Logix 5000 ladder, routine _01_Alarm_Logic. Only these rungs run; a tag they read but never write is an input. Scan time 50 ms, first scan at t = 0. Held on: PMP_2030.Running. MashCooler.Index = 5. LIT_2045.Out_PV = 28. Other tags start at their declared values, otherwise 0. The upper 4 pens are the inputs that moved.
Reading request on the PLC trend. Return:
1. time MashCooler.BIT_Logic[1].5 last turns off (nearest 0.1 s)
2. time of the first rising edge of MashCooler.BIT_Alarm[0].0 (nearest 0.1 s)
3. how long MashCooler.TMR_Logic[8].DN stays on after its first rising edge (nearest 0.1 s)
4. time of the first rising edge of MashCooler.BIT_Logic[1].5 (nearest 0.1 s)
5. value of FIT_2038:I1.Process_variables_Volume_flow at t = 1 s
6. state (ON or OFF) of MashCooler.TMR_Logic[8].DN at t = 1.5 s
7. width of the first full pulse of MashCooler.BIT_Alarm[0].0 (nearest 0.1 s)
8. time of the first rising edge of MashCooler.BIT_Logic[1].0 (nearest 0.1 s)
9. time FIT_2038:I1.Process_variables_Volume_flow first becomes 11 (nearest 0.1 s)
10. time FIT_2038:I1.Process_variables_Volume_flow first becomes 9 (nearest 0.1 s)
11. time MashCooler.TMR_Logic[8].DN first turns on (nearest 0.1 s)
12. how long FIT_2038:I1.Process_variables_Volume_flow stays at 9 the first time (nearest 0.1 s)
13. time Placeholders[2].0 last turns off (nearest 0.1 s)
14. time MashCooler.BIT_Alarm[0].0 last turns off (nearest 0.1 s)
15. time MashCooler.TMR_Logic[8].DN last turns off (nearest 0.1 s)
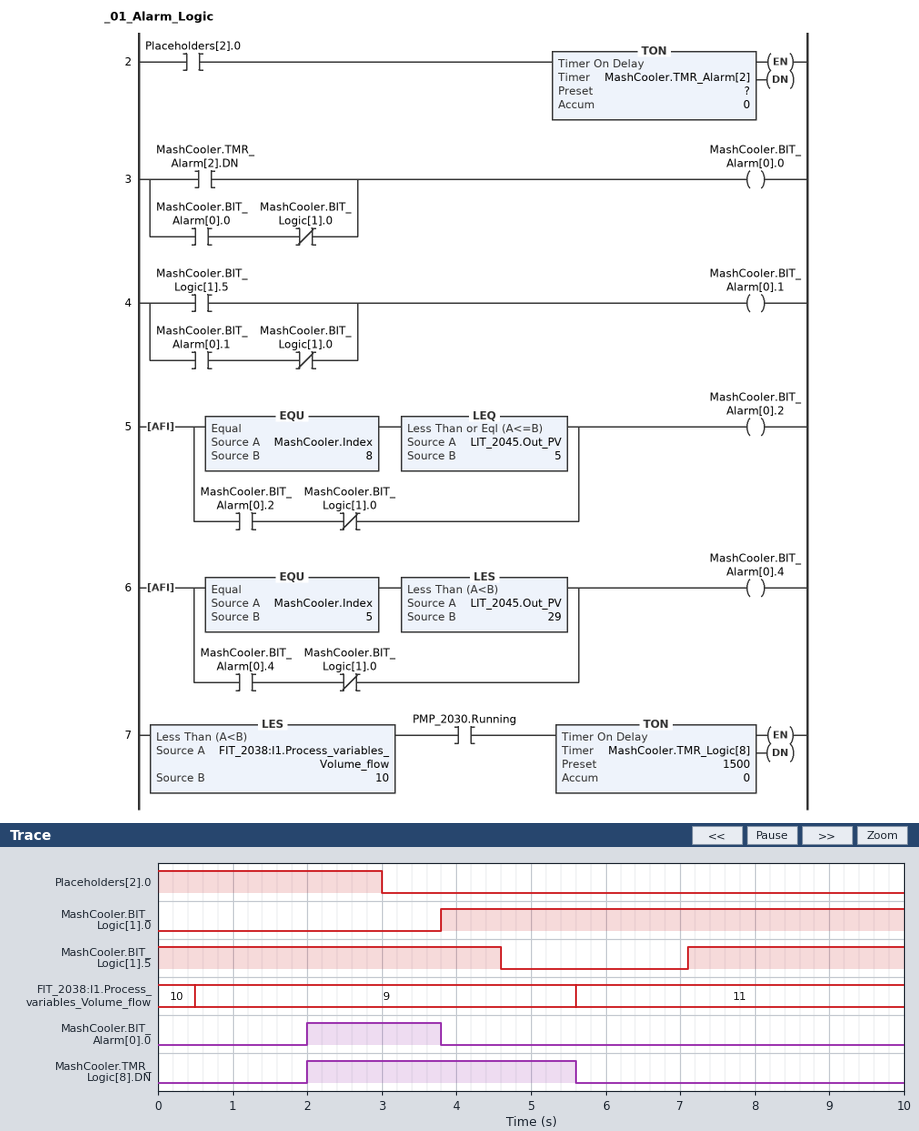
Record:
4.6 s
2.0 s
3.6 s
7.1 s
9
OFF
1.8 s
3.8 s
5.6 s
0.5 s
2.0 s
5.1 s
3.0 s
3.8 s
5.6 s
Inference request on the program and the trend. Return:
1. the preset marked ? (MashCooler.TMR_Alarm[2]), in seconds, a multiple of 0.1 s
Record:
2.0 s
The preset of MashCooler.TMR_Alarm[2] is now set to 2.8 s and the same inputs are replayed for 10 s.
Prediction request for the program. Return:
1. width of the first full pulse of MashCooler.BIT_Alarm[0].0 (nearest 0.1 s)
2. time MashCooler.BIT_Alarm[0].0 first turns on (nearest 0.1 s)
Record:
1.0 s
2.8 s
